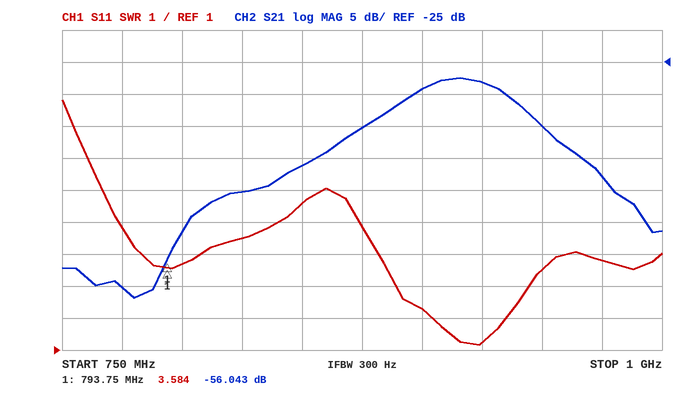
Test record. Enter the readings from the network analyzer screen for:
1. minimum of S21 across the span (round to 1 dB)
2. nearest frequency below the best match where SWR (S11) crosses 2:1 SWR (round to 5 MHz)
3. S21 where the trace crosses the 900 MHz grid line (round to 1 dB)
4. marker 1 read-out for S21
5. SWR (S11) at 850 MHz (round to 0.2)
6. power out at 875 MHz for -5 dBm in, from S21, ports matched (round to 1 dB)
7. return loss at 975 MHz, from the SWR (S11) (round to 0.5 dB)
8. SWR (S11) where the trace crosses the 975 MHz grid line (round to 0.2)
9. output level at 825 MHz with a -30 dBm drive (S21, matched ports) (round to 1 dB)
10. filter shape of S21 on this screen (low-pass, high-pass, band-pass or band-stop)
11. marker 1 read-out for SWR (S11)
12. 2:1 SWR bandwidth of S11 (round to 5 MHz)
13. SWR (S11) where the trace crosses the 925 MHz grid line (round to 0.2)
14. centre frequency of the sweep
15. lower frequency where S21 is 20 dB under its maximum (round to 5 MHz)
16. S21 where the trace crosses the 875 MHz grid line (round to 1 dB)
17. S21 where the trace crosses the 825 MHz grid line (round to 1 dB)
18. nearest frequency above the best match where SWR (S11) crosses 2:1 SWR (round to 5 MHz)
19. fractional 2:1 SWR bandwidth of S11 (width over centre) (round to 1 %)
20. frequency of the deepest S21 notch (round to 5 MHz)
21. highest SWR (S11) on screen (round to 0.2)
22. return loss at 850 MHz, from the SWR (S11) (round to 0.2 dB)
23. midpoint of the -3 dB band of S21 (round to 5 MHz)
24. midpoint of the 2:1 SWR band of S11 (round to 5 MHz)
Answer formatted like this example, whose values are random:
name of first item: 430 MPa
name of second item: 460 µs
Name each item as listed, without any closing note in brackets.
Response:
minimum of S21 across the span: -62 dB
nearest frequency below the best match where SWR (S11) crosses 2:1 SWR: 905 MHz
S21 where the trace crosses the 900 MHz grid line: -29 dB
marker 1 read-out for S21: -56.043 dB
SWR (S11) at 850 MHz: 5.6
power out at 875 MHz for -5 dBm in, from S21, ports matched: -40 dBm
return loss at 975 MHz, from the SWR (S11): 4.5 dB
SWR (S11) where the trace crosses the 975 MHz grid line: 3.8
output level at 825 MHz with a -30 dBm drive (S21, matched ports): -75 dBm
filter shape of S21 on this screen: band-pass
marker 1 read-out for SWR: 3.584
2:1 SWR bandwidth of S11: 30 MHz
SWR (S11) where the trace crosses the 925 MHz grid line: 1.2
centre frequency of the sweep: 875 MHz
lower frequency where S21 is 20 dB under its maximum: 810 MHz
S21 where the trace crosses the 875 MHz grid line: -35 dB
S21 where the trace crosses the 825 MHz grid line: -45 dB
nearest frequency above the best match where SWR (S11) crosses 2:1 SWR: 935 MHz
fractional 2:1 SWR bandwidth of S11 (width over centre): 3 %
frequency of the deepest S21 notch: 780 MHz
highest SWR (S11) on screen: 8.8
return loss at 850 MHz, from the SWR (S11): 3.2 dB
midpoint of the -3 dB band of S21: 915 MHz
midpoint of the 2:1 SWR band of S11: 920 MHz
